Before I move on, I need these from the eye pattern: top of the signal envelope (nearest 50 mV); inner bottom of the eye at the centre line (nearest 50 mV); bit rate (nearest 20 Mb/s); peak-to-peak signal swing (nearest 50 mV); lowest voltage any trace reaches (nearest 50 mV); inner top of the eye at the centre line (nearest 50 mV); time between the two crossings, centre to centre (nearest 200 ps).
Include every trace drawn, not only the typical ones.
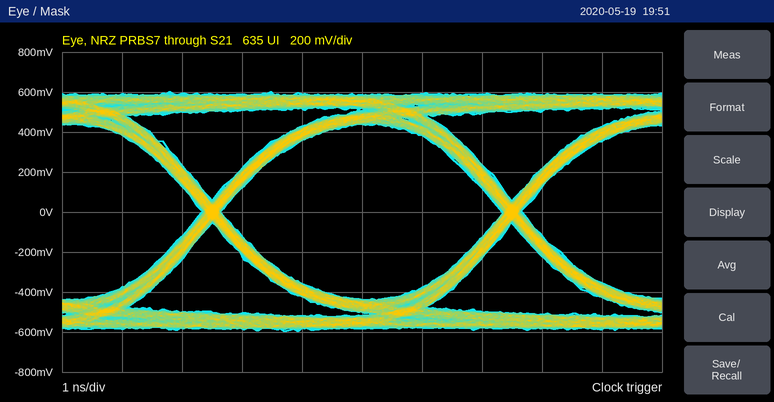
600 mV
-450 mV
200 Mb/s
1.20 V
-600 mV
450 mV
5.0 ns
